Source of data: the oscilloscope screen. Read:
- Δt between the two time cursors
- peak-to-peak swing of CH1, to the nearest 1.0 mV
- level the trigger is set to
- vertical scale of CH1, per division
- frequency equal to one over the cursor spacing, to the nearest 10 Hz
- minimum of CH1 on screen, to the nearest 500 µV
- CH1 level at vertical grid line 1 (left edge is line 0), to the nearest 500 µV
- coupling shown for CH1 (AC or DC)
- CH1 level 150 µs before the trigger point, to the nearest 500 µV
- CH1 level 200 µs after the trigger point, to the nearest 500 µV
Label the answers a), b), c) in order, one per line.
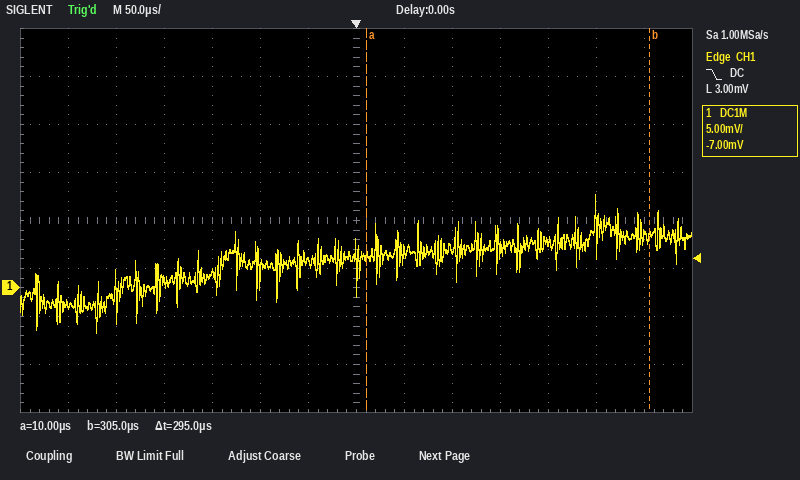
a) 295 µs
b) 14.0 mV
c) 3.00 mV
d) 5 mV
e) 3.39 kHz
f) -4.5 mV
g) -1.5 mV
h) DC
i) 1.5 mV
j) 5.0 mV
